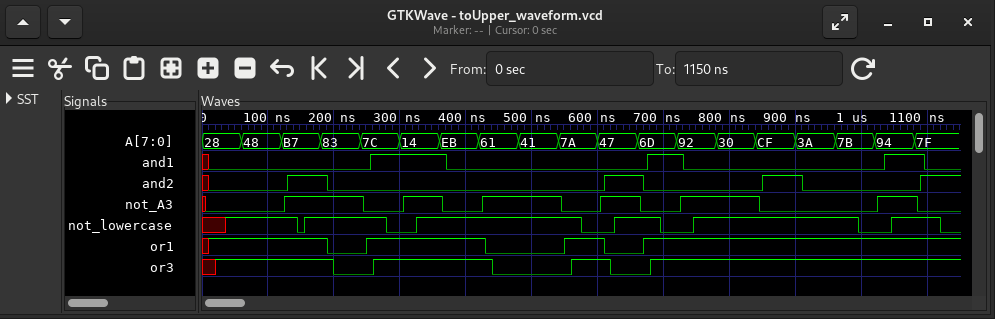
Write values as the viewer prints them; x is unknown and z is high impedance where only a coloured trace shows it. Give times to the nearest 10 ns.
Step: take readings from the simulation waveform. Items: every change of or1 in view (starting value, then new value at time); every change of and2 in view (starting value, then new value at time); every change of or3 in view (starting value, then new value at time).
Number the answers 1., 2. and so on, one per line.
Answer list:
1. x, 1 at 10 ns, 0 at 190 ns, 1 at 250 ns, 0 at 430 ns, 1 at 550 ns, 0 at 610 ns, 1 at 670 ns
2. x, 0 at 10 ns, 1 at 130 ns, 0 at 190 ns, 1 at 610 ns, 0 at 670 ns, 1 at 850 ns, 0 at 910 ns, 1 at 1090 ns
3. x, 1 at 20 ns, 0 at 200 ns, 1 at 260 ns, 0 at 440 ns, 1 at 560 ns, 0 at 620 ns, 1 at 680 ns
